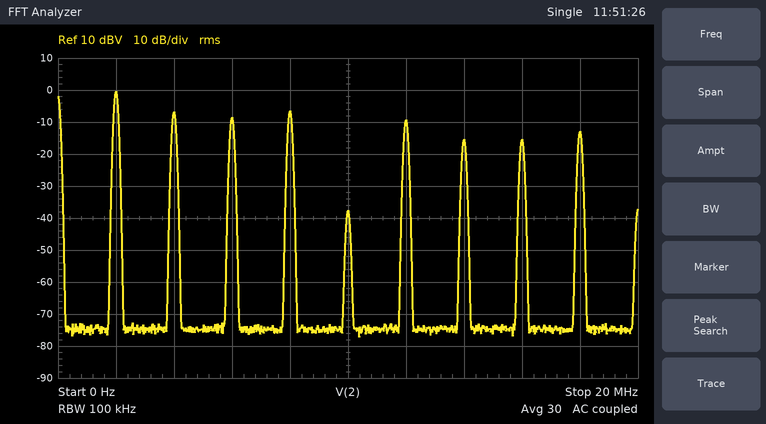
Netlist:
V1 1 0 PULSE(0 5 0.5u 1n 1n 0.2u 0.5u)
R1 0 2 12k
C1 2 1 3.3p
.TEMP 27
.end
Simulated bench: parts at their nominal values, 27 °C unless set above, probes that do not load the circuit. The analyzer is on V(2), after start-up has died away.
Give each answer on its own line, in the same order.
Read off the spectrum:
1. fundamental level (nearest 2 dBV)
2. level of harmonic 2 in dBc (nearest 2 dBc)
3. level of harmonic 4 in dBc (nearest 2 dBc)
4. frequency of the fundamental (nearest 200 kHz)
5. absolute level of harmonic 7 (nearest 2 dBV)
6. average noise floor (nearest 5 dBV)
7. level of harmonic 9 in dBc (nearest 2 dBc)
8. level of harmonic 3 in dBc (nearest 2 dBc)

0 dBV
-6 dBc
-6 dBc
2.0 MHz
-16 dBV
-75 dBV
-12 dBc
-8 dBc
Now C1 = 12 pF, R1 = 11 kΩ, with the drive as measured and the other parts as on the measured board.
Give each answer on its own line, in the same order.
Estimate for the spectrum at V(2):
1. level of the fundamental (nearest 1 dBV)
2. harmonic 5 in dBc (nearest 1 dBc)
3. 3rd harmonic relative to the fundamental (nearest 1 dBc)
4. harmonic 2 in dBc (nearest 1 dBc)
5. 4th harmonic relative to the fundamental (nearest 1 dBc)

5 dBV
-42 dBc
-12 dBc
-9 dBc
-11 dBc
